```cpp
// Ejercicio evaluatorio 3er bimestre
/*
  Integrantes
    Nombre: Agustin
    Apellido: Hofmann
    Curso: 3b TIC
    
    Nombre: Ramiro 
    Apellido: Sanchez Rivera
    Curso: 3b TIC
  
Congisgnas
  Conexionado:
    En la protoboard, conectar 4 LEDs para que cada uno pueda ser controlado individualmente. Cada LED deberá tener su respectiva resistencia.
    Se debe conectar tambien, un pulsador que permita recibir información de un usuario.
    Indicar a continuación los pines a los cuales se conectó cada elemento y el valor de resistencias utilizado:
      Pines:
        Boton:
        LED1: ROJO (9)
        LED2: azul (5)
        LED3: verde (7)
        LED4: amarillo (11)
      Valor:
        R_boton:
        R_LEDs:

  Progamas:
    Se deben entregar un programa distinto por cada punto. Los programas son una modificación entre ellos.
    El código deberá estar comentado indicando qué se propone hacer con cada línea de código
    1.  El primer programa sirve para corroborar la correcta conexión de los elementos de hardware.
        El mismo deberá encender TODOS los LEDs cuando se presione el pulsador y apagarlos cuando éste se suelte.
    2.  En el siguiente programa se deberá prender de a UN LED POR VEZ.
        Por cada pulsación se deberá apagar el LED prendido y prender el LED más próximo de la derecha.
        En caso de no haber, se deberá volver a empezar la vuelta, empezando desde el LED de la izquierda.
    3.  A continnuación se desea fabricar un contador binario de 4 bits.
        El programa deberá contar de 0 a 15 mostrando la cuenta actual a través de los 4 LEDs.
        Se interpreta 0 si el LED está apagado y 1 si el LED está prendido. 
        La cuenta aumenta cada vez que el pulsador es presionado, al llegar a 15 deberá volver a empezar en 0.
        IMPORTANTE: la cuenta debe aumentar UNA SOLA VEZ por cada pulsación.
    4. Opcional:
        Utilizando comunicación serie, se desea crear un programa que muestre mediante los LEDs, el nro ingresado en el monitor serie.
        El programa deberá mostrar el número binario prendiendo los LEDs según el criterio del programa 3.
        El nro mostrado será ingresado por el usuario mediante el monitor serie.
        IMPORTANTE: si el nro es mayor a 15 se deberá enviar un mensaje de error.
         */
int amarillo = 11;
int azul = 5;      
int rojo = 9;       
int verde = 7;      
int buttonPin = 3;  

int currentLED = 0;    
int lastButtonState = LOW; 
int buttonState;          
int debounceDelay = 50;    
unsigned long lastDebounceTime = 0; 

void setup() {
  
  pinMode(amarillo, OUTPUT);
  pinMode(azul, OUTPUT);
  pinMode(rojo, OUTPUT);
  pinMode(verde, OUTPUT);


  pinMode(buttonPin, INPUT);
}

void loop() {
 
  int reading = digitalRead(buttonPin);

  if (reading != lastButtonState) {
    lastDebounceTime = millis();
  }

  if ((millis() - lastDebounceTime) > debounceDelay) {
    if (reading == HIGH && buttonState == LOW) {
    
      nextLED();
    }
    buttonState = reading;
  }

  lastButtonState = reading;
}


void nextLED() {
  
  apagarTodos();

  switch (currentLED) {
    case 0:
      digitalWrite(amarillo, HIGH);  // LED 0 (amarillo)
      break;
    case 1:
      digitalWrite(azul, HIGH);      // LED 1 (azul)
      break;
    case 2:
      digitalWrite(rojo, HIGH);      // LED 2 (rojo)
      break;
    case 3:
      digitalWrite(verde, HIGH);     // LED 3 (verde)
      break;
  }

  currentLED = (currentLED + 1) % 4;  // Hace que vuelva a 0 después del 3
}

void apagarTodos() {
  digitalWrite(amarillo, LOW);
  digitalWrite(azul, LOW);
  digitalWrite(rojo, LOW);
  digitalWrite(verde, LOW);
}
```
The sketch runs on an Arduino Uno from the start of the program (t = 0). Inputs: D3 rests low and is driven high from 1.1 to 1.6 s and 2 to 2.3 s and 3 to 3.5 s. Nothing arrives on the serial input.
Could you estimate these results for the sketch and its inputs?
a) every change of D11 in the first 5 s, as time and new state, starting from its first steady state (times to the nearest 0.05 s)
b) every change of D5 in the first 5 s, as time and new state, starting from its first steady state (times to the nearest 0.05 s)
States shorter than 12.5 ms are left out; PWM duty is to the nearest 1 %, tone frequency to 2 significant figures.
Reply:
0 s low; 1.15 s high; 2.05 s low
0 s low; 2.05 s high; 3.05 s low
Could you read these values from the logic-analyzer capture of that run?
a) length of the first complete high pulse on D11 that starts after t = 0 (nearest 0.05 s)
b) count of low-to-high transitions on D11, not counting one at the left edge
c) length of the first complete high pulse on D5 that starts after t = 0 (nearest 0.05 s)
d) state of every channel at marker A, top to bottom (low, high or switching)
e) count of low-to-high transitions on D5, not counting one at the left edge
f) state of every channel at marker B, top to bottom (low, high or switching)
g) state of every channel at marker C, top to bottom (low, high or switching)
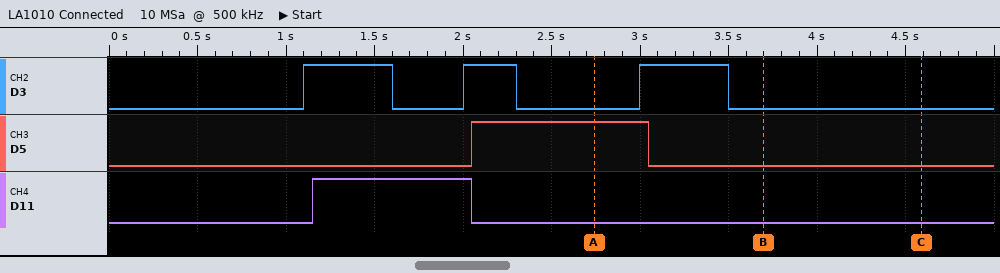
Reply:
0.90 s
1
1.00 s
D3 low, D5 high, D11 low
1
D3 low, D5 low, D11 low
D3 low, D5 low, D11 low
